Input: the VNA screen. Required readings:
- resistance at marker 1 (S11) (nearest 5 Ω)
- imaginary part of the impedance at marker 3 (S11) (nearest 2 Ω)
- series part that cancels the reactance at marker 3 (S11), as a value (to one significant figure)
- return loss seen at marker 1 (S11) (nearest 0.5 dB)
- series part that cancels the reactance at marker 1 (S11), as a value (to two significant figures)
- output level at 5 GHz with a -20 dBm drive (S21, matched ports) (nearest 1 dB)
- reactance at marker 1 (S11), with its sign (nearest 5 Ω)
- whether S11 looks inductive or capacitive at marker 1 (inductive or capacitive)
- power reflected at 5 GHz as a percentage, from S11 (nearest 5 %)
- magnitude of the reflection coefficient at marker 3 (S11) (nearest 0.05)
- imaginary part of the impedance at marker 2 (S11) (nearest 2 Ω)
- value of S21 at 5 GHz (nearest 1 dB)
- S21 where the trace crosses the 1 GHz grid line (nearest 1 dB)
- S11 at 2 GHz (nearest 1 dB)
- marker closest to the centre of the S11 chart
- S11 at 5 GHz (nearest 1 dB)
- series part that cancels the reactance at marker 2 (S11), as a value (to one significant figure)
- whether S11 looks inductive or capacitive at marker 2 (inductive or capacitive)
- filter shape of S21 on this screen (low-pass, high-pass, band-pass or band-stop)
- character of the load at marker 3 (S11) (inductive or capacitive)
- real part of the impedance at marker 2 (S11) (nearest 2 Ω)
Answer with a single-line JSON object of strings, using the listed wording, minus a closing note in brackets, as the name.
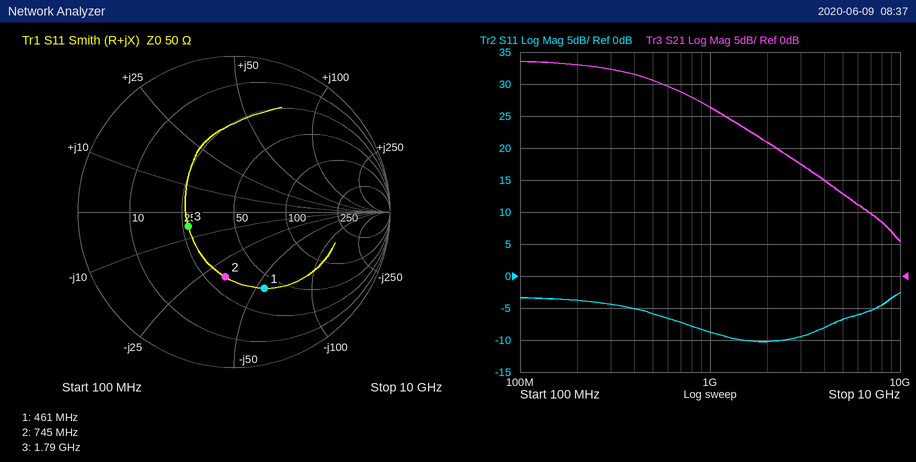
{"resistance at marker 1 (S11)": "40 Ω", "imaginary part of the impedance at marker 3 (S11)": "-6 Ω", "series part that cancels the reactance at marker 3 (S11), as a value": "500 pH", "return loss seen at marker 1 (S11)": "5.5 dB", "series part that cancels the reactance at marker 1 (S11), as a value": "19 nH", "output level at 5 GHz with a -20 dBm drive (S21, matched ports)": "-7 dBm", "reactance at marker 1 (S11), with its sign": "-55 Ω", "whether S11 looks inductive or capacitive at marker 1": "capacitive", "power reflected at 5 GHz as a percentage, from S11": "20 %", "magnitude of the reflection coefficient at marker 3 (S11)": "0.30", "imaginary part of the impedance at marker 2 (S11)": "-32 Ω", "value of S21 at 5 GHz": "13 dB", "S21 where the trace crosses the 1 GHz grid line": "26 dB", "S11 at 2 GHz": "-10 dB", "marker closest to the centre of the S11 chart": "marker 3", "S11 at 5 GHz": "-7 dB", "series part that cancels the reactance at marker 2 (S11), as a value": "7 nH", "whether S11 looks inductive or capacitive at marker 2": "capacitive", "filter shape of S21 on this screen": "low-pass", "character of the load at marker 3 (S11)": "capacitive", "real part of the impedance at marker 2 (S11)": "32 Ω"}
